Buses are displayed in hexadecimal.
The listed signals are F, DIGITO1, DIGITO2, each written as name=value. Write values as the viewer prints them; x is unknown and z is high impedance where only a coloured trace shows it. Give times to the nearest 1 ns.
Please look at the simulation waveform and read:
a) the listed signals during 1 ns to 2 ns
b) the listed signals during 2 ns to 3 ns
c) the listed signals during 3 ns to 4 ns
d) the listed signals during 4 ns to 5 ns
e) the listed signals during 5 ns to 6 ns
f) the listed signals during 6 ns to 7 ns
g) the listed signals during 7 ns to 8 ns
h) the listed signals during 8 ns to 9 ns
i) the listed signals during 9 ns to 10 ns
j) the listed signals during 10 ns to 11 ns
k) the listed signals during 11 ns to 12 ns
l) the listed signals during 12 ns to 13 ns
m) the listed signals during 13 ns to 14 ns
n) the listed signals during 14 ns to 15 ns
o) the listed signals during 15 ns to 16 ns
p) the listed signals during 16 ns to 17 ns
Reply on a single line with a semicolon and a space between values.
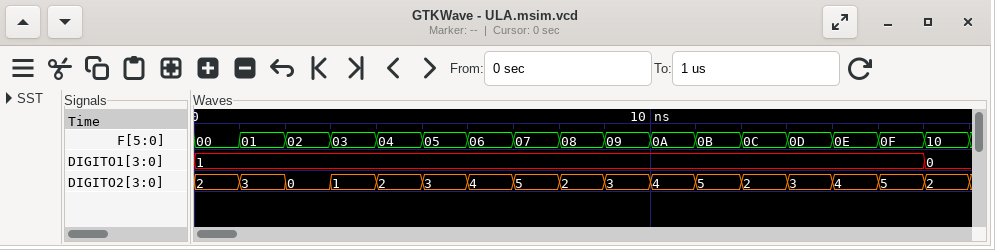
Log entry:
F=01, DIGITO1=1, DIGITO2=3; F=02, DIGITO1=1, DIGITO2=0; F=03, DIGITO1=1, DIGITO2=1; F=04, DIGITO1=1, DIGITO2=2; F=05, DIGITO1=1, DIGITO2=3; F=06, DIGITO1=1, DIGITO2=4; F=07, DIGITO1=1, DIGITO2=5; F=08, DIGITO1=1, DIGITO2=2; F=09, DIGITO1=1, DIGITO2=3; F=0A, DIGITO1=1, DIGITO2=4; F=0B, DIGITO1=1, DIGITO2=5; F=0C, DIGITO1=1, DIGITO2=2; F=0D, DIGITO1=1, DIGITO2=3; F=0E, DIGITO1=1, DIGITO2=4; F=0F, DIGITO1=1, DIGITO2=5; F=10, DIGITO1=0, DIGITO2=2
